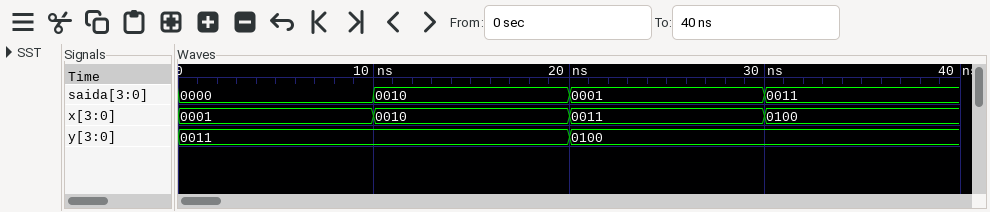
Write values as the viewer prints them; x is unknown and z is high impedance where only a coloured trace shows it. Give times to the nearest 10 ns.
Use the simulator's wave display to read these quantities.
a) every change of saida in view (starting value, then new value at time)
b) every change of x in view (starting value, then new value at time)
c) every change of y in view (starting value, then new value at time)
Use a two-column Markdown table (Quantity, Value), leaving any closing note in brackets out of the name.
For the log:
| Quantity | Value |
|---|---|
| every change of saida in view | 0000, 0010 at 10 ns, 0001 at 20 ns, 0011 at 30 ns |
| every change of x in view | 0001, 0010 at 10 ns, 0011 at 20 ns, 0100 at 30 ns |
| every change of y in view | 0011, 0100 at 20 ns |
